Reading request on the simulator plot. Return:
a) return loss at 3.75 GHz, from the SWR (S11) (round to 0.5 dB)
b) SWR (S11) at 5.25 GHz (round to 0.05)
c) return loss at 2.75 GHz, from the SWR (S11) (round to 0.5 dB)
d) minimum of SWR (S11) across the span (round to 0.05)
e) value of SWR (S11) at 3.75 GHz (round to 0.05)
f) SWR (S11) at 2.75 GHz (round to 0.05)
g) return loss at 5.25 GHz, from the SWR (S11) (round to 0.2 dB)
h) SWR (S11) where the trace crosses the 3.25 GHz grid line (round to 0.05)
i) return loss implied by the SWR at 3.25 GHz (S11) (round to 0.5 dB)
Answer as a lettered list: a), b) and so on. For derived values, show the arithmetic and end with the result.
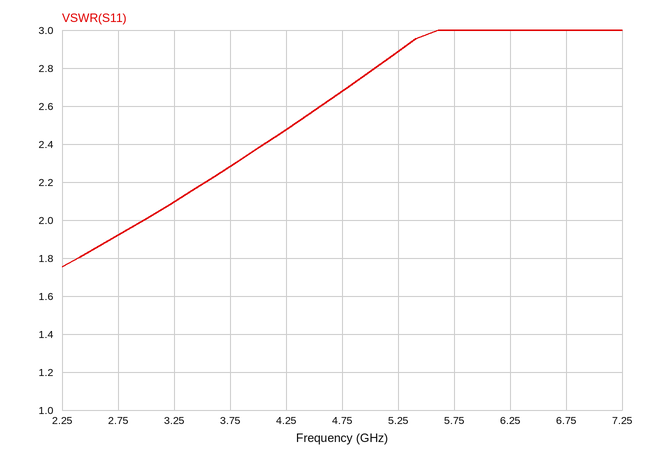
a) −20 log10((2.3 − 1)/(2.3 + 1)) ≈ 8.09 dB, so 8.0 dB to the nearest 0.5 dB
b) 2.90
c) −20 log10((1.9 − 1)/(1.9 + 1)) ≈ 10.2 dB, so 10.0 dB to the nearest 0.5 dB
d) 1.75
e) 2.30
f) 1.90
g) −20 log10((2.9 − 1)/(2.9 + 1)) ≈ 6.2 dB
h) 2.10
i) −20 log10((2.1 − 1)/(2.1 + 1)) ≈ 9.0 dB
